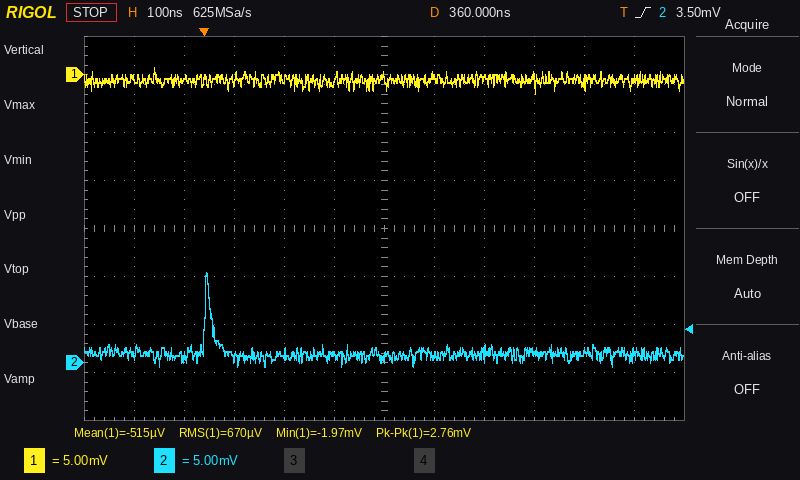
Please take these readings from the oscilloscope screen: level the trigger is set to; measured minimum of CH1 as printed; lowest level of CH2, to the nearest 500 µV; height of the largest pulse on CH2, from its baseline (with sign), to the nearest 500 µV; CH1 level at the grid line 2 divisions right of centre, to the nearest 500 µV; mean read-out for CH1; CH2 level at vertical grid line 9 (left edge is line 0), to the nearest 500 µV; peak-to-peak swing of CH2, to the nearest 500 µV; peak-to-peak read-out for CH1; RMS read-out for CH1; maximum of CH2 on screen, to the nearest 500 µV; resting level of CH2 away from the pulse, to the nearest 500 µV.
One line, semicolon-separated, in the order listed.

3.50 mV; -1.97 mV; -500 µV; +8.5 mV; -500 µV; -515 µV; 1.0 mV; 10.0 mV; 2.76 mV; 670 µV; 9.5 mV; 1.0 mV
